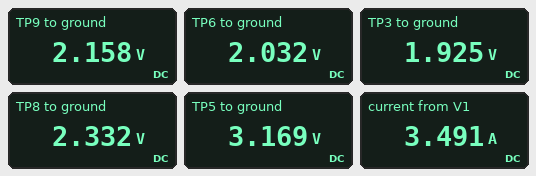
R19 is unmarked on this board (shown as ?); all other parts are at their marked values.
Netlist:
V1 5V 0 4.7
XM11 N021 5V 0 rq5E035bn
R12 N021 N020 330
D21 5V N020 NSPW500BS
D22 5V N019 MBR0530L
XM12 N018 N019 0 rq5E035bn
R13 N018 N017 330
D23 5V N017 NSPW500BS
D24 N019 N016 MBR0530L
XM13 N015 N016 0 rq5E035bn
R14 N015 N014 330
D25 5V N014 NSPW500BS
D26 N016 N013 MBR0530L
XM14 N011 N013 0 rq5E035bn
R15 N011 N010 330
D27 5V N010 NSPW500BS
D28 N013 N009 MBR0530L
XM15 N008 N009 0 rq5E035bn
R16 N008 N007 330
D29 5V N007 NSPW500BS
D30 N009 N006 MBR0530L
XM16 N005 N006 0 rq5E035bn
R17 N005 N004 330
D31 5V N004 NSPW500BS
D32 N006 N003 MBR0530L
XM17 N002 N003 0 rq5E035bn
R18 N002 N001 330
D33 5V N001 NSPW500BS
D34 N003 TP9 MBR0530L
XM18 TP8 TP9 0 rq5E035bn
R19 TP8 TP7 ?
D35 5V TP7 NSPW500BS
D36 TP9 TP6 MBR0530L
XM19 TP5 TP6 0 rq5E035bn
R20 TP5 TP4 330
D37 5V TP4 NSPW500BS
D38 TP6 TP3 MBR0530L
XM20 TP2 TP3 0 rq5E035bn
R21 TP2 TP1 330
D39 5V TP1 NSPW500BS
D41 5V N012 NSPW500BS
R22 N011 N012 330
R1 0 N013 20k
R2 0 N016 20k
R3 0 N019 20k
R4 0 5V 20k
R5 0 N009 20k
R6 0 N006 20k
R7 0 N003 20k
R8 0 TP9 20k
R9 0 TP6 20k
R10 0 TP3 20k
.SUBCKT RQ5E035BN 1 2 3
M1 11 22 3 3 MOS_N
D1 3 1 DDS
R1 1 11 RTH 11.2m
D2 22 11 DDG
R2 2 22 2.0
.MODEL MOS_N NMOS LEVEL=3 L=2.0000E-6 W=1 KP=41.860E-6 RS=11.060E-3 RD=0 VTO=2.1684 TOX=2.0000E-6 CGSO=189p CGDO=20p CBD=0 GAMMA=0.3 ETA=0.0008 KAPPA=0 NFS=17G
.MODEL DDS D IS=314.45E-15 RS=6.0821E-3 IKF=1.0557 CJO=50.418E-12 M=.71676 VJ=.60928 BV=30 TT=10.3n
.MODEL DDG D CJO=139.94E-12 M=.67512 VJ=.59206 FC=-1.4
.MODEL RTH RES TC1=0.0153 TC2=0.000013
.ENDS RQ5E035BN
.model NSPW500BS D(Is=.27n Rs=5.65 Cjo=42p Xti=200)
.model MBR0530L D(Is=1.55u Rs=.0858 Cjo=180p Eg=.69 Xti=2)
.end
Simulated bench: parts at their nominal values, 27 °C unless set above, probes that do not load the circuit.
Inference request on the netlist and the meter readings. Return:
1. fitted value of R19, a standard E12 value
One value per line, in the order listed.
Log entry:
100 Ω
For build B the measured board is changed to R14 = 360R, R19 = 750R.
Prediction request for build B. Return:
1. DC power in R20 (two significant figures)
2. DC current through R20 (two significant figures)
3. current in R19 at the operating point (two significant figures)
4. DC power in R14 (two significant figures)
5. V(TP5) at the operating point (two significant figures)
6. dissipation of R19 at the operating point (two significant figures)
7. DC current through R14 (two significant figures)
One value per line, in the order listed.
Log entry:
700 µW
1.5 mA
3.8 mA
19 mW
3.8 V
11 mW
7.3 mA
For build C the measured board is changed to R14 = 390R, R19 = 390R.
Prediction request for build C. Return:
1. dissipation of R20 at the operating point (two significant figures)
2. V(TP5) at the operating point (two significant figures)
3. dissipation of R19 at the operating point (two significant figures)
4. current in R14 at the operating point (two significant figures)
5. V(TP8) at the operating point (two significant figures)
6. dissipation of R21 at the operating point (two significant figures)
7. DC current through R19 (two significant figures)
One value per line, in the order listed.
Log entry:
1.1 mW
3.7 V
20 mW
6.7 mA
1.4 V
59 µW
7.1 mA
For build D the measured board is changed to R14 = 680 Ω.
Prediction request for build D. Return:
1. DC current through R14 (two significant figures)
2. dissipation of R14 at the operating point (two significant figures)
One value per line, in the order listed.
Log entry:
3.9 mA
10 mW
